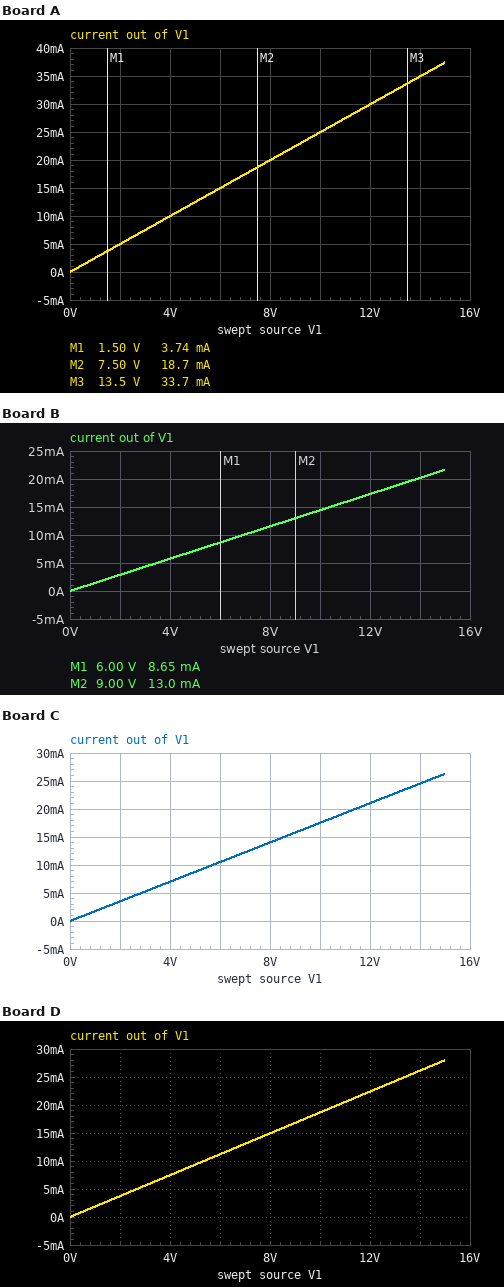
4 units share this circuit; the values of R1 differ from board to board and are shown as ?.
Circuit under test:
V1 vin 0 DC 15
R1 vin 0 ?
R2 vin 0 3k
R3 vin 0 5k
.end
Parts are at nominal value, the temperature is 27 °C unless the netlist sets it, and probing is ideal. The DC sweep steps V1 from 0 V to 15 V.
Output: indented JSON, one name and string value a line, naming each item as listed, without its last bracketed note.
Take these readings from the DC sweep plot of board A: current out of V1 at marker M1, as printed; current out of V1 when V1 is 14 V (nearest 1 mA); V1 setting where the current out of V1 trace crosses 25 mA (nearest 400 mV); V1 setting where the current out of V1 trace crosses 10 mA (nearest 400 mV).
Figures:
{
  "current out of V1 at marker M1, as printed": "3.74 mA",
  "current out of V1 when V1 is 14 V": "35 mA",
  "V1 setting where the current out of V1 trace crosses 25 mA": "10.0 V",
  "V1 setting where the current out of V1 trace crosses 10 mA": "4.0 V"
}
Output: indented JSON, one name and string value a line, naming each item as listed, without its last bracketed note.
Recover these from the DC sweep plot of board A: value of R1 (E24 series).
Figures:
{
  "value of R1": "510 Ω"
}
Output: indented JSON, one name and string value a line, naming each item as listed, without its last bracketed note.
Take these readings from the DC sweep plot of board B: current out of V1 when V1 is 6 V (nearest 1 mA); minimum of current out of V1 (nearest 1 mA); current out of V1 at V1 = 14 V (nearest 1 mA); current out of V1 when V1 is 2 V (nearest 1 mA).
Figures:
{
  "current out of V1 when V1 is 6 V": "9 mA",
  "minimum of current out of V1": "0 A",
  "current out of V1 at V1 = 14 V": "20 mA",
  "current out of V1 when V1 is 2 V": "3 mA"
}
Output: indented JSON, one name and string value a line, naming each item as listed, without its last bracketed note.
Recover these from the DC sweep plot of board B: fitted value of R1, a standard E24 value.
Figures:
{
  "fitted value of R1, a standard E24 value": "1.1 kΩ"
}
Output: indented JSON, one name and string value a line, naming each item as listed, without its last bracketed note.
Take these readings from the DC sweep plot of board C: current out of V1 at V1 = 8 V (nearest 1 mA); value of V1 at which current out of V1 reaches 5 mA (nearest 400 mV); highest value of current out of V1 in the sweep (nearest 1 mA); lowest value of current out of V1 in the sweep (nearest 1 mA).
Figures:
{
  "current out of V1 at V1 = 8 V": "14 mA",
  "value of V1 at which current out of V1 reaches 5 mA": "2.8 V",
  "highest value of current out of V1 in the sweep": "26 mA",
  "lowest value of current out of V1 in the sweep": "0 A"
}
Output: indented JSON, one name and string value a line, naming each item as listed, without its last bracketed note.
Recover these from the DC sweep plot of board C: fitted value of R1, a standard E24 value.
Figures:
{
  "fitted value of R1, a standard E24 value": "820 Ω"
}
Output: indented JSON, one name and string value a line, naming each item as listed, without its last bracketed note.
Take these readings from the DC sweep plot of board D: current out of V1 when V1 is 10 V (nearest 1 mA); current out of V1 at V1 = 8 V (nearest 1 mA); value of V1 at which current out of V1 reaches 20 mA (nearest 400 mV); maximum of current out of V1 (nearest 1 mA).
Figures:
{
  "current out of V1 when V1 is 10 V": "19 mA",
  "current out of V1 at V1 = 8 V": "15 mA",
  "value of V1 at which current out of V1 reaches 20 mA": "10.8 V",
  "maximum of current out of V1": "28 mA"
}
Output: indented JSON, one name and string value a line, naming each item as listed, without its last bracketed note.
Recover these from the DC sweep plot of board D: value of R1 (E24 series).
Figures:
{
  "value of R1": "750 Ω"
}
